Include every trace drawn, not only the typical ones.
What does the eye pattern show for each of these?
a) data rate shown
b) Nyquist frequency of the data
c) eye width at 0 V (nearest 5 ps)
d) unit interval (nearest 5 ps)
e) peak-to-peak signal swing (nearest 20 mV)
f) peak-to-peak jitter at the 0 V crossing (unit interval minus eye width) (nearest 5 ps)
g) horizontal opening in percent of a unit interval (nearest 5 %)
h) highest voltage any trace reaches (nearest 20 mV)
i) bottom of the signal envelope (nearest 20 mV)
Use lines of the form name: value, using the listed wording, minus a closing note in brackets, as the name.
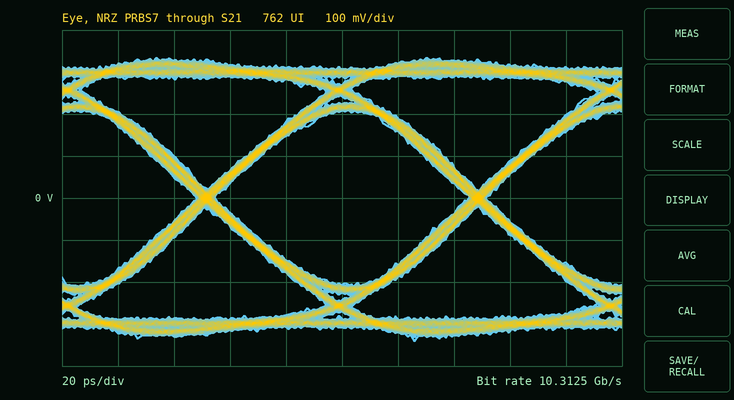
data rate shown: 10.3125 Gb/s
Nyquist frequency of the data: 5.15625 GHz
eye width at 0 V: 90 ps
unit interval: 95 ps
peak-to-peak signal swing: 680 mV
peak-to-peak jitter at the 0 V crossing (unit interval minus eye width): 5 ps
horizontal opening in percent of a unit interval: 95 %
highest voltage any trace reaches: 340 mV
bottom of the signal envelope: -340 mV
